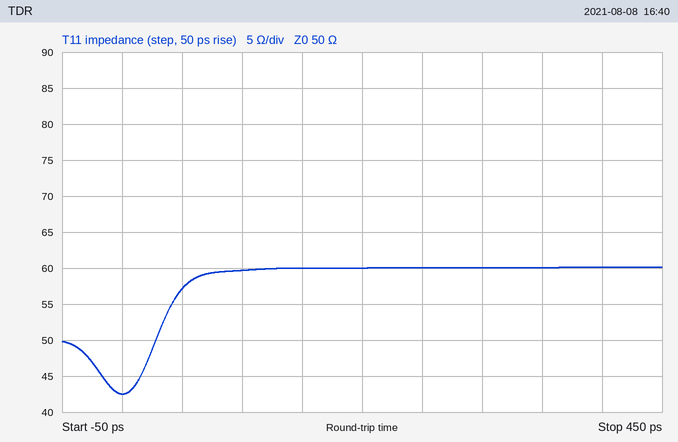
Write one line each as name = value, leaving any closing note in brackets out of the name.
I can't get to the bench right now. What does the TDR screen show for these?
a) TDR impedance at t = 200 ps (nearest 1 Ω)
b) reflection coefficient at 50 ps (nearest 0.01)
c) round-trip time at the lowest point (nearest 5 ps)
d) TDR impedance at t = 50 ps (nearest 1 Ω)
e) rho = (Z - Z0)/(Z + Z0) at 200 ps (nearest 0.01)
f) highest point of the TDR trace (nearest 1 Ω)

TDR impedance at t = 200 ps = 60 Ω
reflection coefficient at 50 ps = +0.07
round-trip time at the lowest point = 0 ps
TDR impedance at t = 50 ps = 57 Ω
rho = (Z - Z0)/(Z + Z0) at 200 ps = +0.09
highest point of the TDR trace = 60 Ω
